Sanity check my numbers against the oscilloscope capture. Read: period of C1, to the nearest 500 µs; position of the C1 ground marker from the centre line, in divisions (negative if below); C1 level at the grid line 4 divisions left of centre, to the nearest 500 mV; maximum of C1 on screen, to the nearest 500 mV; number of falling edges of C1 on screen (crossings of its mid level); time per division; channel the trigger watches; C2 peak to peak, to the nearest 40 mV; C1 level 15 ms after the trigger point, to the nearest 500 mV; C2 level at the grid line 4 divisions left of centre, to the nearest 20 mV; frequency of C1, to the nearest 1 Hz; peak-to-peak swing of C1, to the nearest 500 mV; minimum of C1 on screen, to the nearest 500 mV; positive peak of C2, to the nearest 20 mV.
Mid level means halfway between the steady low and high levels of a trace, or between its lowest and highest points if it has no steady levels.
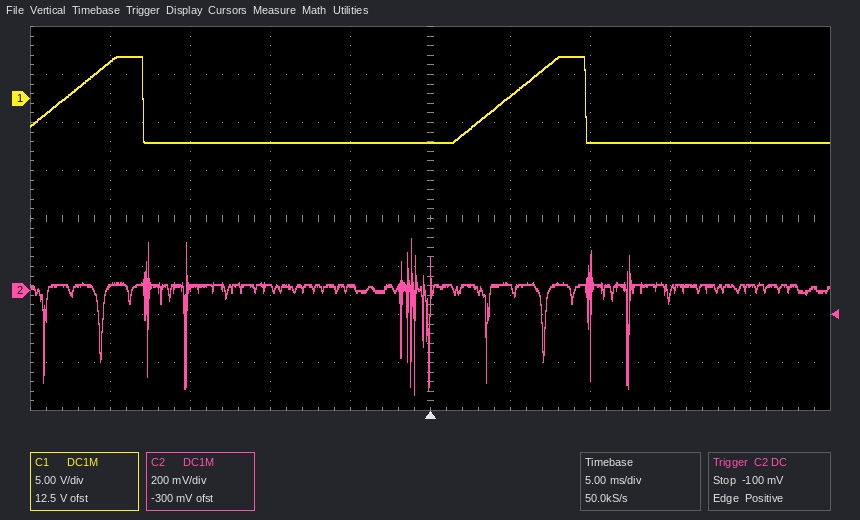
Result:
27.5 ms
+2.5 div
4.0 V
4.5 V
2
5 ms
C2
640 mV
-4.5 V
20 mV
36 Hz
9.0 V
-4.5 V
220 mV
